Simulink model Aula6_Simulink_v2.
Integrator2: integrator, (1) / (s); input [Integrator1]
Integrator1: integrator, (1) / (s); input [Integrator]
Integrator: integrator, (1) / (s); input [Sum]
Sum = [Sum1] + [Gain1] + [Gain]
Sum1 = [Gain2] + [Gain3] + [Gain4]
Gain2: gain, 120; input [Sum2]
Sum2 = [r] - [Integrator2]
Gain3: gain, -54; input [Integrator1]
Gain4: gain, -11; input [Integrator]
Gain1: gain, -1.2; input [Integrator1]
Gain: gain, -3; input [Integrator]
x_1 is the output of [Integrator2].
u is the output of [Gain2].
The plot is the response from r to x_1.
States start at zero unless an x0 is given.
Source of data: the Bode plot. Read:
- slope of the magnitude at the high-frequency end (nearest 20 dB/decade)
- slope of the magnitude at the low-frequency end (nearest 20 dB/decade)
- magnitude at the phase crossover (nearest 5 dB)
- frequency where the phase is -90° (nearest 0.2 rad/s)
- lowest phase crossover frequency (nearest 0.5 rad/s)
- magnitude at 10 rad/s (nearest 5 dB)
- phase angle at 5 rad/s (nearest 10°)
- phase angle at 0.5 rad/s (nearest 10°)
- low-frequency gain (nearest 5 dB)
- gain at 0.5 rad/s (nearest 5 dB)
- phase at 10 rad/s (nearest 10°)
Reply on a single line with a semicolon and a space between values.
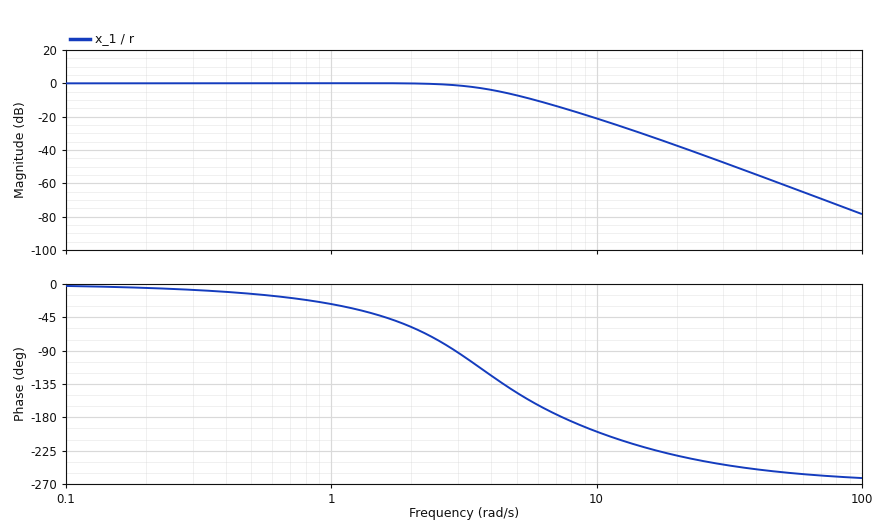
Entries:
-60 dB/decade; 0 dB/decade; -15 dB; 3.0 rad/s; 7.5 rad/s; -20 dB; -150°; -10°; 0 dB; 0 dB; -200°
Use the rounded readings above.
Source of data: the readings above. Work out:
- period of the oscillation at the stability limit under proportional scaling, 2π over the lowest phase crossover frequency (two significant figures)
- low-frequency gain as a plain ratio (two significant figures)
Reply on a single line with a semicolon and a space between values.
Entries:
0.84 s; 1.0
